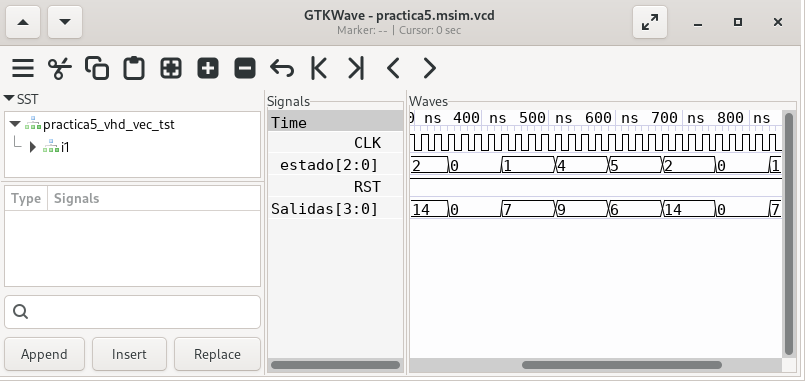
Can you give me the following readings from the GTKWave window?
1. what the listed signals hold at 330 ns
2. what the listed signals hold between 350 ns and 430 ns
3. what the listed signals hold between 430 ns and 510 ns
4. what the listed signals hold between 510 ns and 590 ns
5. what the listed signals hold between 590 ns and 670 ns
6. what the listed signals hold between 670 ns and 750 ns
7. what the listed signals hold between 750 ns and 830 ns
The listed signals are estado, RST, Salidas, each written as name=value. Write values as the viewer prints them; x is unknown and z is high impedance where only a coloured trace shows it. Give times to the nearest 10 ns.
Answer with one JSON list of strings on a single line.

["estado=2, RST=1, Salidas=14", "estado=0, RST=1, Salidas=0", "estado=1, RST=1, Salidas=7", "estado=4, RST=1, Salidas=9", "estado=5, RST=1, Salidas=6", "estado=2, RST=1, Salidas=14", "estado=0, RST=1, Salidas=0"]
